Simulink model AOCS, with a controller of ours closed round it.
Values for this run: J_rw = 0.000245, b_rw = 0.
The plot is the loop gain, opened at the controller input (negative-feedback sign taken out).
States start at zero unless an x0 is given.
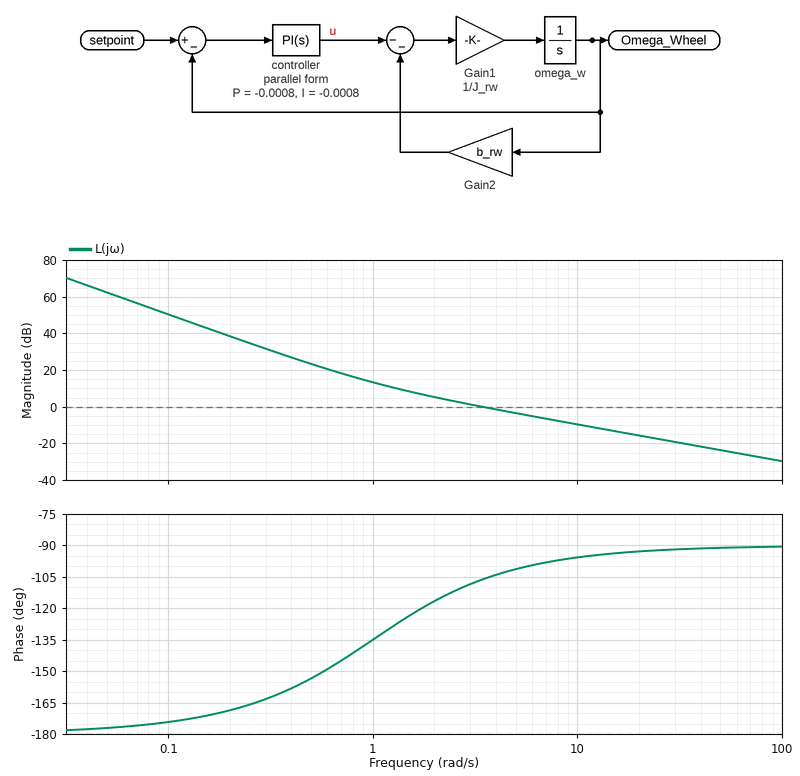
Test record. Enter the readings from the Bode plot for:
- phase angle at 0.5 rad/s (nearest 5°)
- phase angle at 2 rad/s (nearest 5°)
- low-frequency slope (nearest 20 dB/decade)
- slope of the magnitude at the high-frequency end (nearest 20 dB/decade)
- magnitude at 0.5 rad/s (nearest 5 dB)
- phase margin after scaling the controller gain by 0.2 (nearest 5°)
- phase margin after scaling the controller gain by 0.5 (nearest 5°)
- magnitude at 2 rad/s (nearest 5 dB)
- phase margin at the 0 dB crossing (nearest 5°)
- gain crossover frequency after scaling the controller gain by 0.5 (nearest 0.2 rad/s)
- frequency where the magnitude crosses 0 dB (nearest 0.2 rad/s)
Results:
-155°
-115°
-40 dB/decade
-20 dB/decade
25 dB
45°
60°
5 dB
75°
1.8 rad/s
3.4 rad/s
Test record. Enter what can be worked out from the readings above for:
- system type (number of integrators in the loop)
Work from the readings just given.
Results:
2
